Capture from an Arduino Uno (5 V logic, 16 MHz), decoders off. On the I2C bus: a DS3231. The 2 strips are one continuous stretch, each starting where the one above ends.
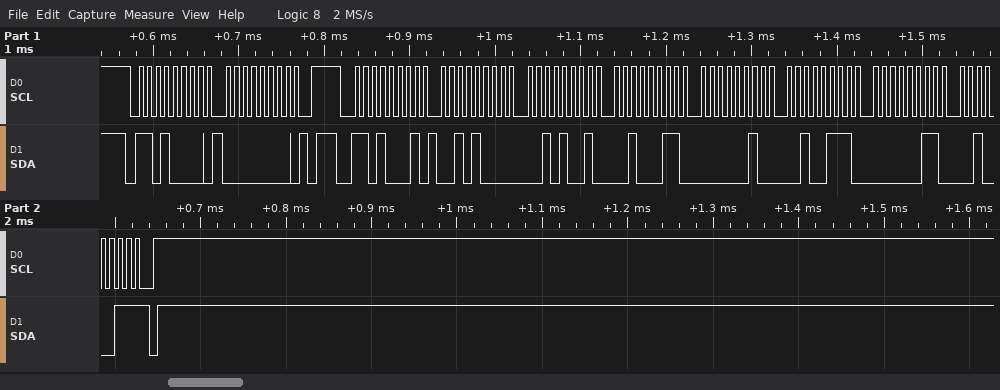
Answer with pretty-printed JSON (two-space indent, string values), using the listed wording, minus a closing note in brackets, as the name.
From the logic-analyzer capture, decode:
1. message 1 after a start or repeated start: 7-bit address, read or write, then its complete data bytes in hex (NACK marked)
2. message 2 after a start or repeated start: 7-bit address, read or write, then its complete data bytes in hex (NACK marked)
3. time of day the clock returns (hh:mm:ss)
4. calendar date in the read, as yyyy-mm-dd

{
  "message 1 after a start or repeated start: 7-bit address, read or write, then its complete data bytes in hex": "0x68 write: 00",
  "message 2 after a start or repeated start: 7-bit address, read or write, then its complete data bytes in hex": "0x68 read: 28 29 23 02 27 03 23 NACK",
  "time of day the clock returns": "23:29:28",
  "calendar date in the read, as yyyy-mm-dd": "2023-03-27"
}
